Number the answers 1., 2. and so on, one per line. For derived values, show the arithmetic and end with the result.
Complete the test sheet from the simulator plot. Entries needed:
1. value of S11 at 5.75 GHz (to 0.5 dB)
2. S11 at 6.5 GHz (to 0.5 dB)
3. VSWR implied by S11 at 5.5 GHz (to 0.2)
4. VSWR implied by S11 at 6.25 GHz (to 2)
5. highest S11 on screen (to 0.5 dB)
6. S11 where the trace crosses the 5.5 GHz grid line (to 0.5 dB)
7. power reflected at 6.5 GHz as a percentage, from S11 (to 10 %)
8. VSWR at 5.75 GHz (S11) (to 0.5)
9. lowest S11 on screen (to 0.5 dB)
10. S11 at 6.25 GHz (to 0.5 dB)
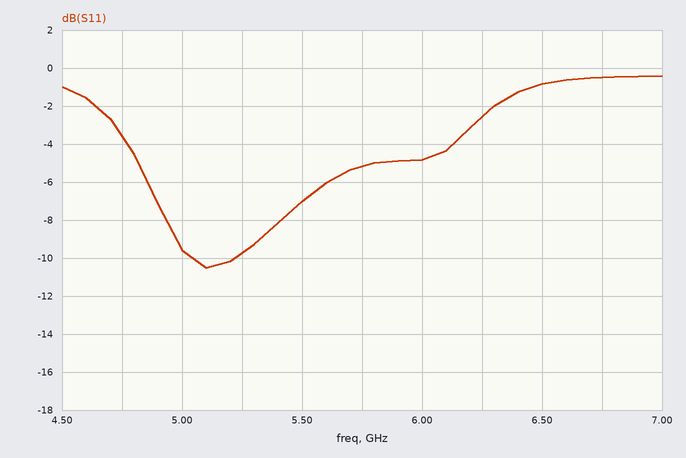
1. -5.0 dB
2. -1.0 dB
3. |Γ| = 10^(-7/20) = 0.4467; VSWR = (1 + 0.4467)/(1 − 0.4467) ≈ 2.6
4. |Γ| = 10^(-2.5/20) = 0.7499; VSWR = (1 + 0.7499)/(1 − 0.7499) ≈ 7.00, so 6 to the nearest 2
5. -0.5 dB
6. -7.0 dB
7. 10^(-1/10) ≈ 79.4 %, so 80 % to the nearest 10 %
8. |Γ| = 10^(-5/20) = 0.5623; VSWR = (1 + 0.5623)/(1 − 0.5623) ≈ 3.57, so 3.5 to the nearest 0.5
9. -10.5 dB
10. -2.5 dB
